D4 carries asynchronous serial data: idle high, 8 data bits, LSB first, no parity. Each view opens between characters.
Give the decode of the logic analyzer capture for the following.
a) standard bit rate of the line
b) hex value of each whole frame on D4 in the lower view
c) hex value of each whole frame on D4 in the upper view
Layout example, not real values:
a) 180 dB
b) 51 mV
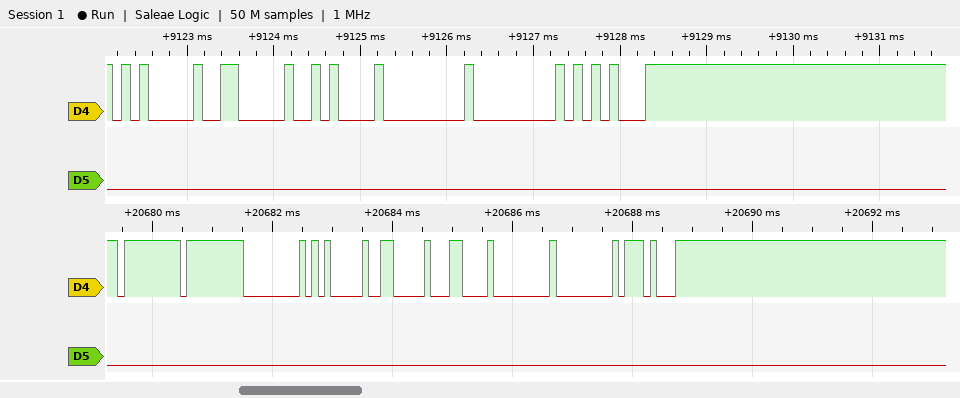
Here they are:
a) 9600 baud
b) FF, FF, 00, 05, 06, 0C, 00, 00, 17
c) 05, 06, 0A, 00, 00, 15
